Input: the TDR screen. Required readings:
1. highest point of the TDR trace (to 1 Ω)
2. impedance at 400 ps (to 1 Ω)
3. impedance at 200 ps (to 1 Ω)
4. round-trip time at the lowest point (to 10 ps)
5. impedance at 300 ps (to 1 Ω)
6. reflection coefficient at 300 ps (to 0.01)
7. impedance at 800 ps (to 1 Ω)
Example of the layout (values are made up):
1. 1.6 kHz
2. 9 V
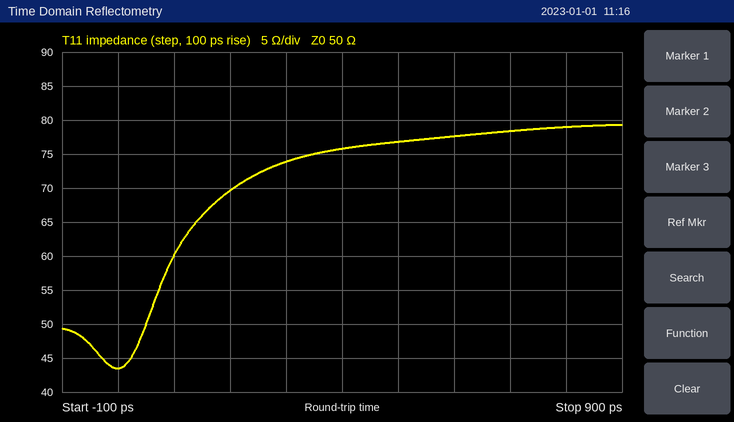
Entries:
1. 79 Ω
2. 76 Ω
3. 70 Ω
4. 0 ps
5. 74 Ω
6. +0.19
7. 79 Ω
